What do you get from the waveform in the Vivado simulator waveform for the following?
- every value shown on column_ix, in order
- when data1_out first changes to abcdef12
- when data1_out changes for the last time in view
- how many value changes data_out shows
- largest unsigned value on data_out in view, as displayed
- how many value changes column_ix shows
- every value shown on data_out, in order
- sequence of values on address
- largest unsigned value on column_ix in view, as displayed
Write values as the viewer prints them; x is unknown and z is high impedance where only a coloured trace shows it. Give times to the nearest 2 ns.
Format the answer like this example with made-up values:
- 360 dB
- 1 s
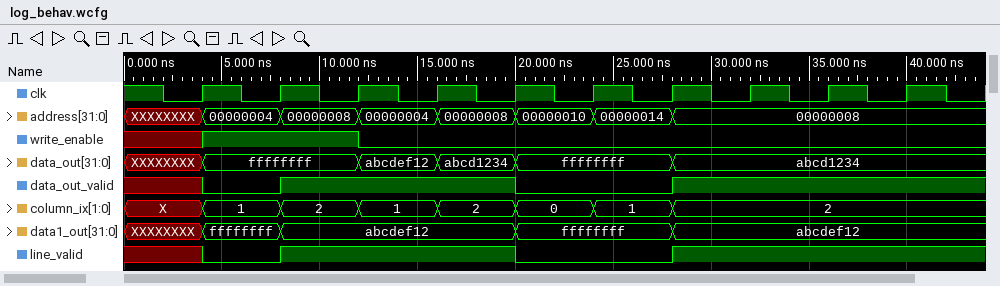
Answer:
- X, 1, 2, 1, 2, 0, 1, 2
- 8 ns
- 28 ns
- 5
- ffffffff
- 7
- XXXXXXXX, ffffffff, abcdef12, abcd1234, ffffffff, abcd1234
- XXXXXXXX, 00000004, 00000008, 00000004, 00000008, 00000010, 00000014, 00000008
- 2
